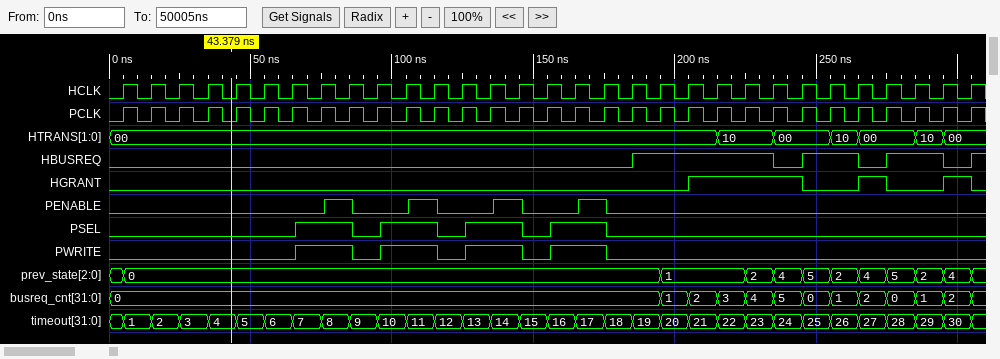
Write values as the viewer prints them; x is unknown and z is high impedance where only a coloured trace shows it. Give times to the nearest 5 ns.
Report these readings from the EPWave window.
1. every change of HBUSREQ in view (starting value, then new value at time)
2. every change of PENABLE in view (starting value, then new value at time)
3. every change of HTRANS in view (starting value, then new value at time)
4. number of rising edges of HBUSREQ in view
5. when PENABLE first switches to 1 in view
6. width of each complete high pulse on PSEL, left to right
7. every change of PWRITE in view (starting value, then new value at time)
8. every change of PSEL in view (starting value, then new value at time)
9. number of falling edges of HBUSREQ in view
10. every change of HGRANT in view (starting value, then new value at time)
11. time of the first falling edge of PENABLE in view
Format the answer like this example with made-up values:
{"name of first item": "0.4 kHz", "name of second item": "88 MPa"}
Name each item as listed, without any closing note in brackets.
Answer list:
{"every change of HBUSREQ in view": "0, 1 at 185 ns, 0 at 235 ns, 1 at 245 ns, 0 at 265 ns, 1 at 275 ns, 0 at 295 ns, 1 at 305 ns", "every change of PENABLE in view": "0, 1 at 75 ns, 0 at 85 ns, 1 at 105 ns, 0 at 115 ns, 1 at 135 ns, 0 at 145 ns, 1 at 165 ns, 0 at 175 ns", "every change of HTRANS in view": "00, 10 at 215 ns, 00 at 235 ns, 10 at 255 ns, 00 at 265 ns, 10 at 285 ns, 00 at 295 ns", "number of rising edges of HBUSREQ in view": "4", "when PENABLE first switches to 1 in view": "75 ns", "width of each complete high pulse on PSEL, left to right": "20 ns, 20 ns, 20 ns, 20 ns", "every change of PWRITE in view": "0, 1 at 65 ns, 0 at 85 ns, 1 at 95 ns, 0 at 115 ns, 1 at 125 ns, 0 at 145 ns, 1 at 155 ns, 0 at 175 ns", "every change of PSEL in view": "0, 1 at 65 ns, 0 at 85 ns, 1 at 95 ns, 0 at 115 ns, 1 at 125 ns, 0 at 145 ns, 1 at 155 ns, 0 at 175 ns", "number of falling edges of HBUSREQ in view": "3", "every change of HGRANT in view": "0, 1 at 205 ns, 0 at 245 ns, 1 at 265 ns, 0 at 275 ns, 1 at 295 ns, 0 at 305 ns", "time of the first falling edge of PENABLE in view": "85 ns"}
